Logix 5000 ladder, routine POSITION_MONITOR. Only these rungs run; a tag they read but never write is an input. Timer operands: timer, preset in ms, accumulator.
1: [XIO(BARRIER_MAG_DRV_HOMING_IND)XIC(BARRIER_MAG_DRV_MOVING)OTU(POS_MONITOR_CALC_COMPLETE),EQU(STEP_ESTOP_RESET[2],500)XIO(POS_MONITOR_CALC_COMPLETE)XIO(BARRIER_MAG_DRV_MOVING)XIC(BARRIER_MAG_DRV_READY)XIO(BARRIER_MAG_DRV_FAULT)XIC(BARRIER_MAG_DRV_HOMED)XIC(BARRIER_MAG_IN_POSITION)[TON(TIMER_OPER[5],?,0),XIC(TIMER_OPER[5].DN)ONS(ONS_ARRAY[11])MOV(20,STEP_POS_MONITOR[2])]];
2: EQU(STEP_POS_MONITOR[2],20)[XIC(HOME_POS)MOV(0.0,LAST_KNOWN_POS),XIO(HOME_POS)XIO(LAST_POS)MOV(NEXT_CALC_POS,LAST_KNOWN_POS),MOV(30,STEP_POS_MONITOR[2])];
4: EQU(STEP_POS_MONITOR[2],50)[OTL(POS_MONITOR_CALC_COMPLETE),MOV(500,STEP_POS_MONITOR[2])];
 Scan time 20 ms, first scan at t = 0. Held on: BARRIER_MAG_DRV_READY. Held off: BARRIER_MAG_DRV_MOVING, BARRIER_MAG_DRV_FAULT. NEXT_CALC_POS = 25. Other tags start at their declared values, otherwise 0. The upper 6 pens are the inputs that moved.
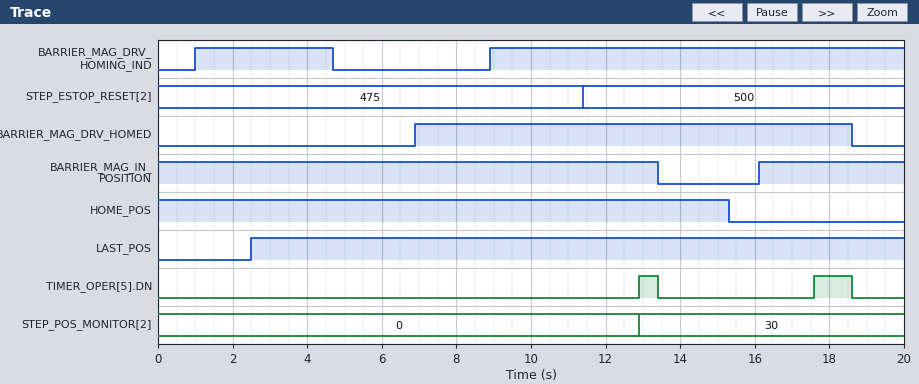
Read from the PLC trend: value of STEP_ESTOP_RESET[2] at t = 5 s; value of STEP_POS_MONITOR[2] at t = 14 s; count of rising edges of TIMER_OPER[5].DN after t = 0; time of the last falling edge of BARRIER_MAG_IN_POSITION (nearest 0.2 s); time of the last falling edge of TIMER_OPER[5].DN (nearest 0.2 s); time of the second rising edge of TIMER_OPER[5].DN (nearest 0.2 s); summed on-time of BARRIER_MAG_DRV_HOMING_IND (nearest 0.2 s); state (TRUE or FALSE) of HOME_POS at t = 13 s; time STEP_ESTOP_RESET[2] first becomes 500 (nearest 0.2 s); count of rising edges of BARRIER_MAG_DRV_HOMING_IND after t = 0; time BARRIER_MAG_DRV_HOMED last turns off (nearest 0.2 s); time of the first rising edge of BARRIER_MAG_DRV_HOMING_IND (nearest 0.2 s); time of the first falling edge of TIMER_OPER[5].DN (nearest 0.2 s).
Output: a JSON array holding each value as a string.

["475", "30", "2", "13.4 s", "18.6 s", "17.6 s", "14.8 s", "TRUE", "11.4 s", "2", "18.6 s", "1.0 s", "13.4 s"]
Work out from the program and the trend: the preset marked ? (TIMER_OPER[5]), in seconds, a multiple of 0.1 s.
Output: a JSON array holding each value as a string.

["1.5 s"]
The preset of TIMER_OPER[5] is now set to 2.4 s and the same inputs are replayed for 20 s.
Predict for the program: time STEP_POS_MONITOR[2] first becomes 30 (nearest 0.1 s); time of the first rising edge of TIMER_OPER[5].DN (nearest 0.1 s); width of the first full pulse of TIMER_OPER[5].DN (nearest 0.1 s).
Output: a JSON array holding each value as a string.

["18.5 s", "18.5 s", "0.1 s"]
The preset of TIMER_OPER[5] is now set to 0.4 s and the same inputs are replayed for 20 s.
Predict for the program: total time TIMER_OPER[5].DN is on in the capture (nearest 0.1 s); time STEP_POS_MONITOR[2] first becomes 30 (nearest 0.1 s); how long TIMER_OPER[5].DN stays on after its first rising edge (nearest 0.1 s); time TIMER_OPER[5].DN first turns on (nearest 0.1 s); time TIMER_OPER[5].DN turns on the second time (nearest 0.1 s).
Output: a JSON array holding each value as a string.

["3.7 s", "11.8 s", "1.6 s", "11.8 s", "16.5 s"]
